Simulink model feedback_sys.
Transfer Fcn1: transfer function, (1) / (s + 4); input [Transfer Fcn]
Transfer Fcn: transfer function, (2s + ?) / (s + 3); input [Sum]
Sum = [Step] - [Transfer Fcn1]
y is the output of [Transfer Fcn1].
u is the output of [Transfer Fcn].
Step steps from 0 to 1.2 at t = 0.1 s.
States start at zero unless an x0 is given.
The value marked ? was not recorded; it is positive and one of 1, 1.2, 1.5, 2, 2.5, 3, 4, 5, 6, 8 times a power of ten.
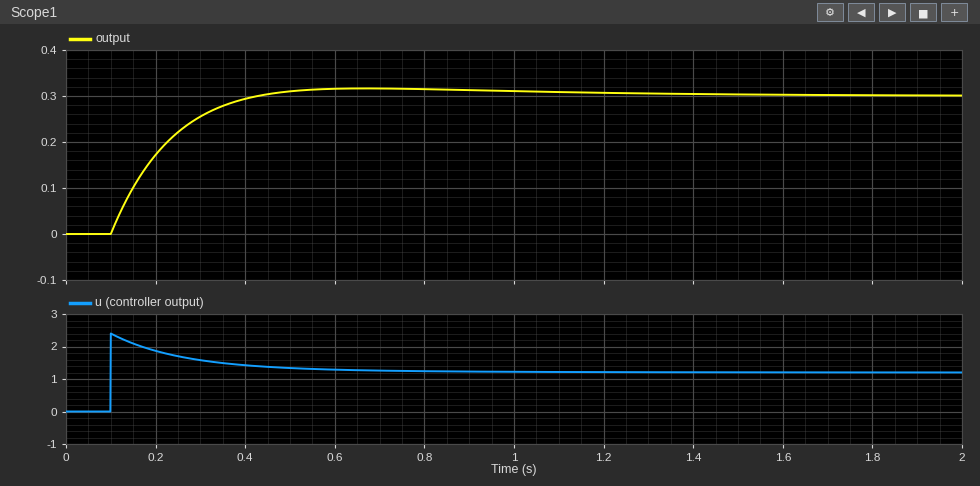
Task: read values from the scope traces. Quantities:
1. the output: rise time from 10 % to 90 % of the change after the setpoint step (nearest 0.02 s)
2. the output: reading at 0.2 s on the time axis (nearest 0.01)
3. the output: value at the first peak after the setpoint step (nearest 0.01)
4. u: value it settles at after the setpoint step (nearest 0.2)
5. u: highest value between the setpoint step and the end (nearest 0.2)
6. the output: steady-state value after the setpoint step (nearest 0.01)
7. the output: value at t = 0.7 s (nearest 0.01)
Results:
0.22 s
0.17
0.32
1.2
2.4
0.30
0.32
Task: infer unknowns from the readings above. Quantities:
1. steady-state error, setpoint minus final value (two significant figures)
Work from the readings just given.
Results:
0.90
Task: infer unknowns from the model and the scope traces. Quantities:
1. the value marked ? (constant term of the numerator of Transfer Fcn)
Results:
4
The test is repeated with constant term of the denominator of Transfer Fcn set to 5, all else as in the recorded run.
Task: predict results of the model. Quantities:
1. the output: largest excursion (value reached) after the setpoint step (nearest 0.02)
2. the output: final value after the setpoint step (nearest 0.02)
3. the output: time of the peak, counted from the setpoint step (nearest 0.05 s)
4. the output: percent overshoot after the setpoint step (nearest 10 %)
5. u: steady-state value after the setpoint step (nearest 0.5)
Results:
0.24
0.20
0.35 s
20 %
1.0
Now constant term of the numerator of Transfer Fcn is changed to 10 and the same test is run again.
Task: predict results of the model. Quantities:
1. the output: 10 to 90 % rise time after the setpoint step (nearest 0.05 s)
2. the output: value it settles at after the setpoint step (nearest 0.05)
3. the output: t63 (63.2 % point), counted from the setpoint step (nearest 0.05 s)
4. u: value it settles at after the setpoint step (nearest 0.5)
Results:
0.45 s
0.55
0.20 s
2.0
